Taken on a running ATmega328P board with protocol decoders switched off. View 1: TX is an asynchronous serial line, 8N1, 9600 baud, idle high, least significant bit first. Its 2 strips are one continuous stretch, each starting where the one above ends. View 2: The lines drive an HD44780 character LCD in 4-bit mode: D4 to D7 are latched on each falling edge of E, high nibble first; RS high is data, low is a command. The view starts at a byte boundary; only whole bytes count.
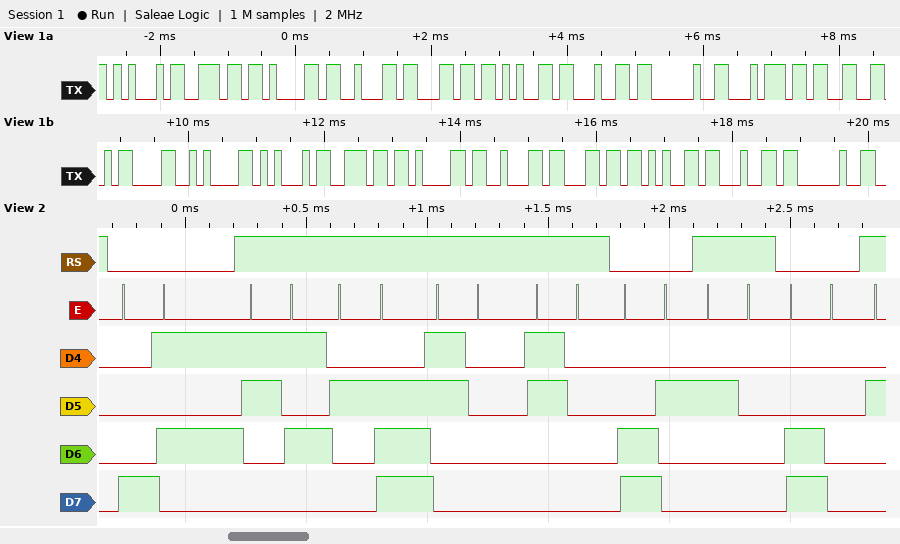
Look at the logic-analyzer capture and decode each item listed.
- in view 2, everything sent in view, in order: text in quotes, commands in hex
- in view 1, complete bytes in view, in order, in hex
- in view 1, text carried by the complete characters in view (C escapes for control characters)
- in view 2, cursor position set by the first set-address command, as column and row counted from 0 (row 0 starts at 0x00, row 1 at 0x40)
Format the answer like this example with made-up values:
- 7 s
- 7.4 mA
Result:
- 0x85 "5.00" 0xC2 " " 0xC0
- 45 6E 61 62 6C 65 64 20 74 33 0D 0A 45 6E 61 62 6C 65 64 20
- "Enabled t3\r\nEnabled "
- column 5, row 0
